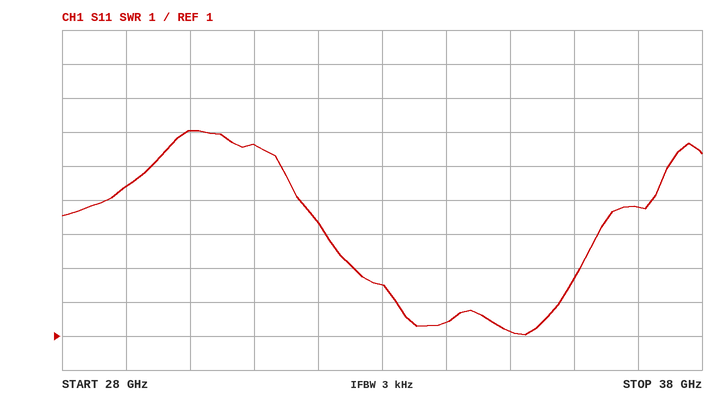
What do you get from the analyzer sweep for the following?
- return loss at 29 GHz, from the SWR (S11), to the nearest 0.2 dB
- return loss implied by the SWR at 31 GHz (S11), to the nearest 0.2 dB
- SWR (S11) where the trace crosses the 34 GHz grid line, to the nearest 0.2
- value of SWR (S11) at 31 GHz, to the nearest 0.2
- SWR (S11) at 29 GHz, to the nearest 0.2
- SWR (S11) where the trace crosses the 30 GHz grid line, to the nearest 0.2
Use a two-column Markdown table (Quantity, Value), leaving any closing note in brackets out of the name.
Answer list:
| Quantity | Value |
|---|---|
| return loss at 29 GHz, from the SWR (S11), to the nearest 0.2 dB | 3.2 dB |
| return loss implied by the SWR at 31 GHz (S11), to the nearest 0.2 dB | 2.6 dB |
| SWR (S11) where the trace crosses the 34 GHz grid line, to the nearest 0.2 | 1.4 |
| value of SWR (S11) at 31 GHz, to the nearest 0.2 | 6.6 |
| SWR (S11) at 29 GHz, to the nearest 0.2 | 5.4 |
| SWR (S11) where the trace crosses the 30 GHz grid line, to the nearest 0.2 | 7.0 |
